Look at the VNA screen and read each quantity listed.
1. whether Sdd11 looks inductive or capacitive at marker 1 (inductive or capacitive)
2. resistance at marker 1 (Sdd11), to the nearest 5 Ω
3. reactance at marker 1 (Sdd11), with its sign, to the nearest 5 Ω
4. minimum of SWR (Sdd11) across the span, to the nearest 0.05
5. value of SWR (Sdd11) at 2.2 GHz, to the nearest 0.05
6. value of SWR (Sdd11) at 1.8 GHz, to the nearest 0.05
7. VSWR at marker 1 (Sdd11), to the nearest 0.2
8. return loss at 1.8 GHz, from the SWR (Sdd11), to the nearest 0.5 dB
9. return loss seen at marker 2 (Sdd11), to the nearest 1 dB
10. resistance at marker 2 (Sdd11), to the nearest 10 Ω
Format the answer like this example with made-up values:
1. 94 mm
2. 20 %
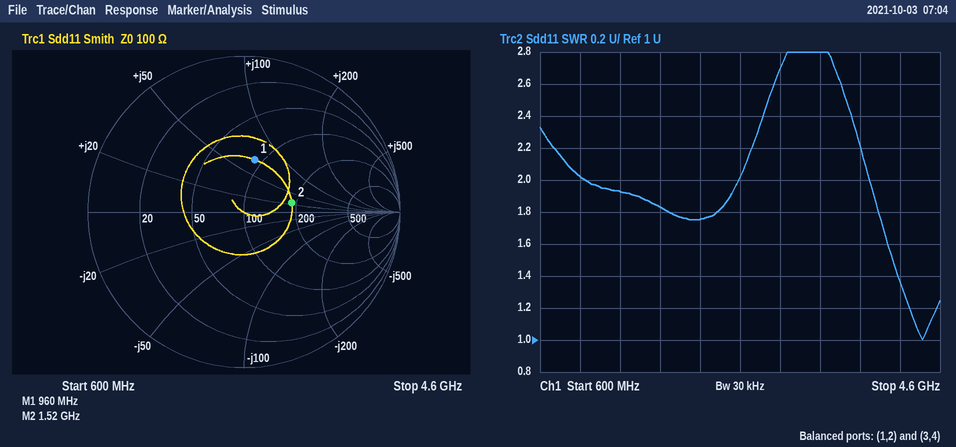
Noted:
1. inductive
2. 90 Ω
3. +70 Ω
4. 1.00
5. 1.75
6. 1.85
7. 2.0
8. 10.5 dB
9. 10 dB
10. 190 Ω
